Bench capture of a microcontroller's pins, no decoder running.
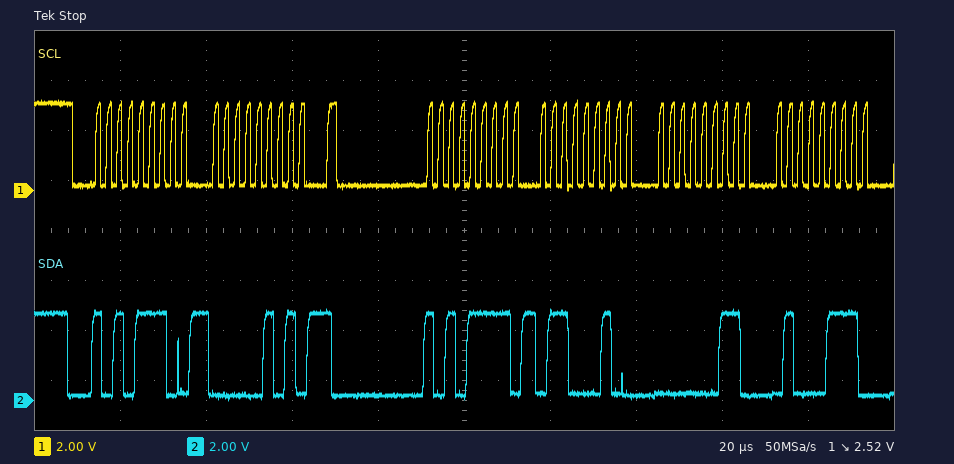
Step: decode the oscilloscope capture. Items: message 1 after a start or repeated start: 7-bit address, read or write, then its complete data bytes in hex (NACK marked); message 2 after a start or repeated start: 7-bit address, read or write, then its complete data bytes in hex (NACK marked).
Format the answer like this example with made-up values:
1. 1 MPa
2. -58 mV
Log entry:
1. 0x57 write: 05
2. 0x57 read: 62 03 47
